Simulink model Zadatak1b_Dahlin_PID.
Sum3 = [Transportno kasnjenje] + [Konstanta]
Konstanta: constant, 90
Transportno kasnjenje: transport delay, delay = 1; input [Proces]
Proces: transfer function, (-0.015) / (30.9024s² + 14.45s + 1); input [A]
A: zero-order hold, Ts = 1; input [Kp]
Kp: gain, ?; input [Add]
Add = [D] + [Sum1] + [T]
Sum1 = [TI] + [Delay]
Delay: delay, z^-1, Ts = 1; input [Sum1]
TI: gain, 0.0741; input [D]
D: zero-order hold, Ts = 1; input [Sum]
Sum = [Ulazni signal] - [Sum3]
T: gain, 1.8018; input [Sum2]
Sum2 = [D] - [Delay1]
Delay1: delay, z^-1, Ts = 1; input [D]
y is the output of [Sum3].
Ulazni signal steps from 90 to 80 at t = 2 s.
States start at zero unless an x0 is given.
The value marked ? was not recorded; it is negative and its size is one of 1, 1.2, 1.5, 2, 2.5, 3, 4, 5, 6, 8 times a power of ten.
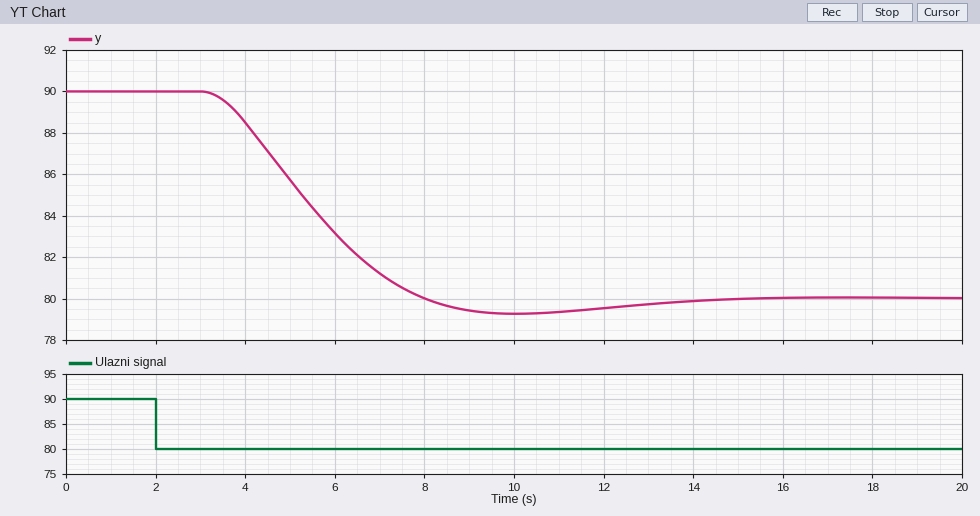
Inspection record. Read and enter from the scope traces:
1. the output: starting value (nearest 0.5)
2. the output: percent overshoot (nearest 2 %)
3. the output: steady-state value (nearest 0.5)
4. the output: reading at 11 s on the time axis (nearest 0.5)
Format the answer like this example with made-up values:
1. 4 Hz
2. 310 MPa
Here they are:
1. 90.0
2. 8 %
3. 80.0
4. 79.5
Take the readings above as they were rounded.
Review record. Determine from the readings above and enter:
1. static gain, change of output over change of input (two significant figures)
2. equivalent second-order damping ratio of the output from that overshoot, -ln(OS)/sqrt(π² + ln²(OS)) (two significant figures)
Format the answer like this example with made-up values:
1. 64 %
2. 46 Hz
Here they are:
1. 1.0
2. 0.63
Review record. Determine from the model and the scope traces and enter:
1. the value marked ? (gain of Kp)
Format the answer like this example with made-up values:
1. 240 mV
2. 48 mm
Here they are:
1. -250
